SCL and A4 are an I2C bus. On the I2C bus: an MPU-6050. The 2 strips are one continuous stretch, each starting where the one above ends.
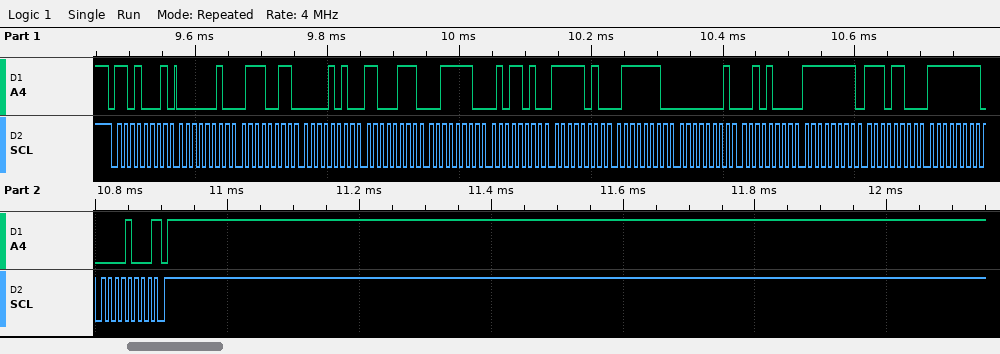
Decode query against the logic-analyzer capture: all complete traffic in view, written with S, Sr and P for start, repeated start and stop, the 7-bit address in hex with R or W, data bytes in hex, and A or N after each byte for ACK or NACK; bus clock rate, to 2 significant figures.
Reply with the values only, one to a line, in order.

S 68R A 02 A 73 A 0A A C7 A 3E A 5A A FA A 7E A 01 A 28 A FF A EC A FF A 08 N P
100 kHz
